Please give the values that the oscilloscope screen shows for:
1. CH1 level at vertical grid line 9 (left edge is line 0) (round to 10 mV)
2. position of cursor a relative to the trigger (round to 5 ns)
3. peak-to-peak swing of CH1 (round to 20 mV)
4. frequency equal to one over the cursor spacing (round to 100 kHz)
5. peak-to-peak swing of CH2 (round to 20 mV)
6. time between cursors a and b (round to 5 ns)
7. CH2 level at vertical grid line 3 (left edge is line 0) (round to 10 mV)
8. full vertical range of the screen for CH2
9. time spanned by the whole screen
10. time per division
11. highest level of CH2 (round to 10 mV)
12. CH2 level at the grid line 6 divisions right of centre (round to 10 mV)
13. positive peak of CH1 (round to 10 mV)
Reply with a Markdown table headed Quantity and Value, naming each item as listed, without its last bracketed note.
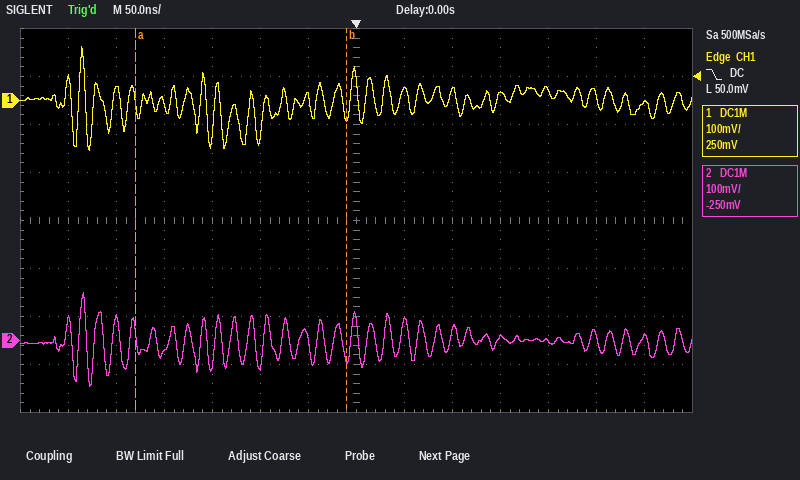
| Quantity | Value |
|---|---|
| CH1 level at vertical grid line 9 (left edge is line 0) | 20 mV |
| position of cursor a relative to the trigger | -230 ns |
| peak-to-peak swing of CH1 | 220 mV |
| frequency equal to one over the cursor spacing | 4.5 MHz |
| peak-to-peak swing of CH2 | 200 mV |
| time between cursors a and b | 220 ns |
| CH2 level at vertical grid line 3 (left edge is line 0) | -20 mV |
| full vertical range of the screen for CH2 | 800 mV |
| time spanned by the whole screen | 700 ns |
| time per division | 50 ns |
| highest level of CH2 | 100 mV |
| CH2 level at the grid line 6 divisions right of centre | 10 mV |
| positive peak of CH1 | 110 mV |
